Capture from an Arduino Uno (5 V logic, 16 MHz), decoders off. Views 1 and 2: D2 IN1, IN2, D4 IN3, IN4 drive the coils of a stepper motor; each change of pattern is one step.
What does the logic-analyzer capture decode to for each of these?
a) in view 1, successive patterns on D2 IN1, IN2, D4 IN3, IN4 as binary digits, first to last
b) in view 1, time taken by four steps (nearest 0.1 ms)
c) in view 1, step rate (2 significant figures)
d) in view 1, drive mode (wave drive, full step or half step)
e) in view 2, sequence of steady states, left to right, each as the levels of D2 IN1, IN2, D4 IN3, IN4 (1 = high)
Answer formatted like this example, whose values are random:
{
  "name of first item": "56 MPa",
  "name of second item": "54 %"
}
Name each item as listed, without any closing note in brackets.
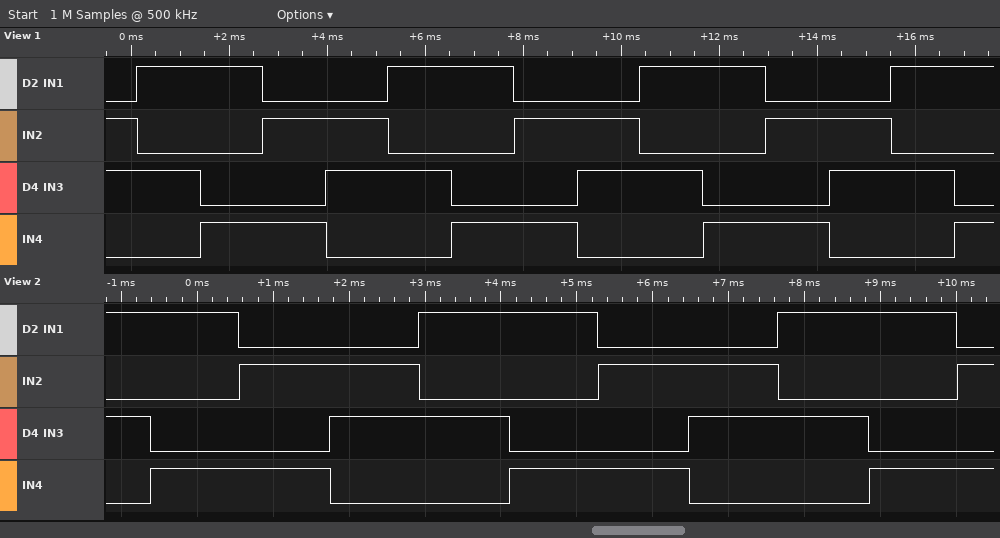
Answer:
{
  "in view 1, successive patterns on D2 IN1, IN2, D4 IN3, IN4 as binary digits, first to last": "0110 1010 1001 0101 0110 1010 1001 0101 0110 1010 1001 0101 0110 1010 1001",
  "in view 1, time taken by four steps": "5.1 ms",
  "in view 1, step rate": "780 steps/s",
  "in view 1, drive mode": "full step",
  "in view 2, sequence of steady states, left to right, each as the levels of D2 IN1, IN2, D4 IN3, IN4": "1010 1001 0101 0110 1010 1001 0101 0110 1010 1001 0101"
}
